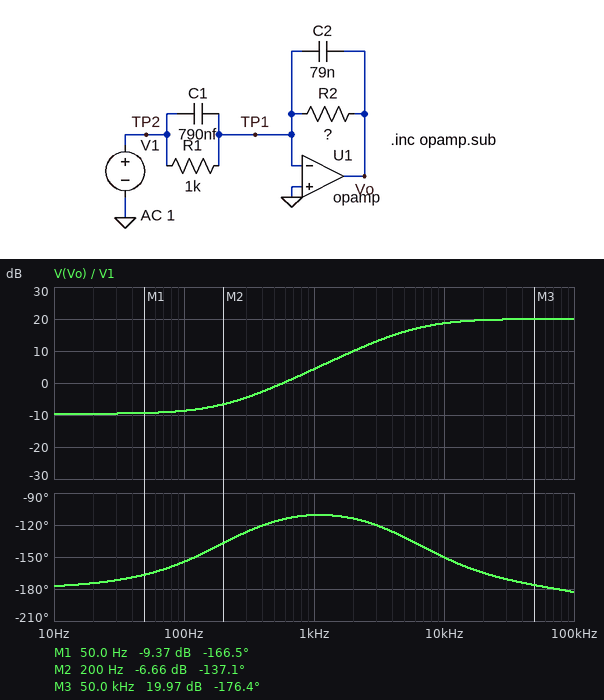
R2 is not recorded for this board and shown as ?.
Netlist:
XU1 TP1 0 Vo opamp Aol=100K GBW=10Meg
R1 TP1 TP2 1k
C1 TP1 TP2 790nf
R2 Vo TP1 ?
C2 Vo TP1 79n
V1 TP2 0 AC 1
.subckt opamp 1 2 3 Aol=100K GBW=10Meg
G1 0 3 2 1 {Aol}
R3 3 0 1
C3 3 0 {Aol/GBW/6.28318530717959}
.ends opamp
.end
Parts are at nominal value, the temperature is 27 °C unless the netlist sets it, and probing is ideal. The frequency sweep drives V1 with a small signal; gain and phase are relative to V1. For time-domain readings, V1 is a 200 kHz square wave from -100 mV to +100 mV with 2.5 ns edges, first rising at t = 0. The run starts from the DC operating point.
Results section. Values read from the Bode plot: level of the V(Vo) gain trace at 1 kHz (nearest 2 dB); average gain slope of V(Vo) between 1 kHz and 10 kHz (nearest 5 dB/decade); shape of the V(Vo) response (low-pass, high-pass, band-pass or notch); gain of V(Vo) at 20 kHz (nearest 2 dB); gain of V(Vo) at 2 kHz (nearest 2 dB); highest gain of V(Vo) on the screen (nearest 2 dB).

4 dB
15 dB/decade
high-pass
20 dB
10 dB
20 dB
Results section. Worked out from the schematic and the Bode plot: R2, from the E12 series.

330 Ω
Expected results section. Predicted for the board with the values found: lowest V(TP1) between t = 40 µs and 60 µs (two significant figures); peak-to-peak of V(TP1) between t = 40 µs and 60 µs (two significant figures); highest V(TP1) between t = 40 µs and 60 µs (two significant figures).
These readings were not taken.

-180 mV
360 mV
180 mV
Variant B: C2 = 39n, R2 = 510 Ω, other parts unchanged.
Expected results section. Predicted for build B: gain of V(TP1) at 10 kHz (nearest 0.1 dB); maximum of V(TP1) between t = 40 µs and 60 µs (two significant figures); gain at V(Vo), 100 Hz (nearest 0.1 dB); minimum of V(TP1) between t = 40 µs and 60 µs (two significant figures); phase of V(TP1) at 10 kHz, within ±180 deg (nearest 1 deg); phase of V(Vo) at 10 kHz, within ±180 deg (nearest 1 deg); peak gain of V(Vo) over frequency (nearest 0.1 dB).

-35.9 dB
190 mV
-4.9 dB
-190 mV
126 deg
-143 deg
26.1 dB
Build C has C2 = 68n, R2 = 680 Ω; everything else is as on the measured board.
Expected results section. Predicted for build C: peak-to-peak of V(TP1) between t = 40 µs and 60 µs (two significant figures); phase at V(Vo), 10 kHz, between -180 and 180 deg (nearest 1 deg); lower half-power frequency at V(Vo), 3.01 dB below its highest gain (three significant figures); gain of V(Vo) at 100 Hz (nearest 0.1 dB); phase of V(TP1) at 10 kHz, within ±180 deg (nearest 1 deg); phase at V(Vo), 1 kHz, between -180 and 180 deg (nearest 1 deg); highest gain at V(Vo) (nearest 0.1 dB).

370 mV
-163 deg
3.41 kHz
-2.4 dB
107 deg
-118 deg
21.3 dB
